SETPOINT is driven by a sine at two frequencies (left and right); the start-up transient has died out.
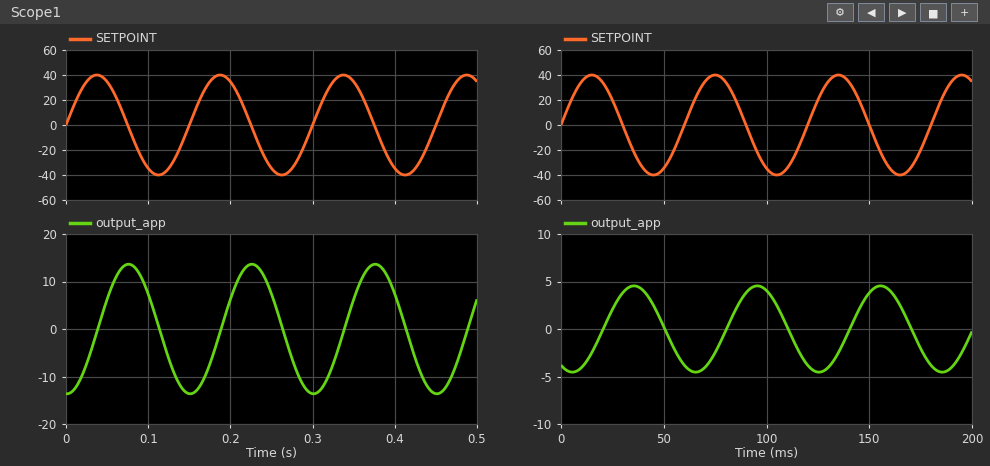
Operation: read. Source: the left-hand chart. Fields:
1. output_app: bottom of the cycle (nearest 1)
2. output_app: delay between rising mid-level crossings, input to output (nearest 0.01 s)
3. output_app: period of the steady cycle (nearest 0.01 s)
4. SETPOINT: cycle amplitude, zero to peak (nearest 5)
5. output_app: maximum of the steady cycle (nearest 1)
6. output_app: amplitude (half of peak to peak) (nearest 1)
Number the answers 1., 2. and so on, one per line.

1. -14
2. 0.04 s
3. 0.15 s
4. 40
5. 14
6. 14
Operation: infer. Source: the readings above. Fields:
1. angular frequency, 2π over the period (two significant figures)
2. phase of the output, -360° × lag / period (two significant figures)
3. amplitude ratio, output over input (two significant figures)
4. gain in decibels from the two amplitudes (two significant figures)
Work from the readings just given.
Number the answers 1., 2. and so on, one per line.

1. 42 rad/s
2. -96°
3. 0.35
4. -9.1 dB
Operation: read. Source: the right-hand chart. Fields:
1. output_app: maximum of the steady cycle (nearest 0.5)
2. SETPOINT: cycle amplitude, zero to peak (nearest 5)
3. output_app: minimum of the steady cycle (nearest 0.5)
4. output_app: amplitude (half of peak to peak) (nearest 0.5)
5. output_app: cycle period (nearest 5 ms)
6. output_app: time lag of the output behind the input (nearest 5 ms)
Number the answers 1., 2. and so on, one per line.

1. 4.5
2. 40
3. -4.5
4. 4.5
5. 60 ms
6. 20 ms
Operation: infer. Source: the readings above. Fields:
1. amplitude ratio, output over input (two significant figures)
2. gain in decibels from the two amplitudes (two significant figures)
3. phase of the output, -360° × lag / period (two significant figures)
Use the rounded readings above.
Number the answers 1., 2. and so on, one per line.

1. 0.11
2. -19 dB
3. -120°
